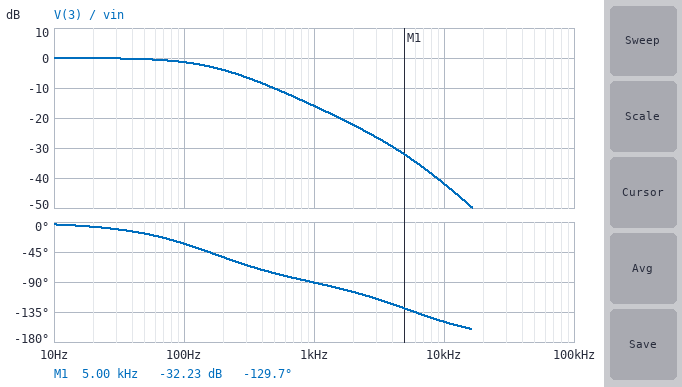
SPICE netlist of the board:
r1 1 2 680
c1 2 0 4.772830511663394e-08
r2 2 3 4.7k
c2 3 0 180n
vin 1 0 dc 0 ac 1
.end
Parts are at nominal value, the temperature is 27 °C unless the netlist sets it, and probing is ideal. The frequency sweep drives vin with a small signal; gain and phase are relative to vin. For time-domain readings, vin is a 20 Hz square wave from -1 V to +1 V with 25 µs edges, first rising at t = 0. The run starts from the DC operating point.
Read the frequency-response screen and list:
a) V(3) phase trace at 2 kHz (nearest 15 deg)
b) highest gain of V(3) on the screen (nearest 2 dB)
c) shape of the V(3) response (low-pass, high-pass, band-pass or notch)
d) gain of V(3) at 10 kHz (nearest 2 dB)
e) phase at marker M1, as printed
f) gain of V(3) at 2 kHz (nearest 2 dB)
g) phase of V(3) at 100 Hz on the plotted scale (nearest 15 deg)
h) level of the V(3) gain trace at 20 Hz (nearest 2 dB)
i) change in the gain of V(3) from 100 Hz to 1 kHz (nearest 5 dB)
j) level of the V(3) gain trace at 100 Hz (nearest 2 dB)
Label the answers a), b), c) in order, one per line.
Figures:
a) -105 deg
b) 0 dB
c) low-pass
d) -42 dB
e) -129.7 deg
f) -22 dB
g) -30 deg
h) 0 dB
i) -15 dB
j) -2 dB
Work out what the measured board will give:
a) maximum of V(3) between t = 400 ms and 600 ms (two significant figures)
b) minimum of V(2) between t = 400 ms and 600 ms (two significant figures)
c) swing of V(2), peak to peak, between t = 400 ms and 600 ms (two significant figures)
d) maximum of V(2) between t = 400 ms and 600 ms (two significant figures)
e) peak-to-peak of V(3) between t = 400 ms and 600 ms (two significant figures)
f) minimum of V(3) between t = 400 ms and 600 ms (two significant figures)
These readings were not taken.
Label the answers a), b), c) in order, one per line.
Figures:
a) 1.0 V
b) -1.0 V
c) 2.0 V
d) 1.0 V
e) 2.0 V
f) -1.0 V
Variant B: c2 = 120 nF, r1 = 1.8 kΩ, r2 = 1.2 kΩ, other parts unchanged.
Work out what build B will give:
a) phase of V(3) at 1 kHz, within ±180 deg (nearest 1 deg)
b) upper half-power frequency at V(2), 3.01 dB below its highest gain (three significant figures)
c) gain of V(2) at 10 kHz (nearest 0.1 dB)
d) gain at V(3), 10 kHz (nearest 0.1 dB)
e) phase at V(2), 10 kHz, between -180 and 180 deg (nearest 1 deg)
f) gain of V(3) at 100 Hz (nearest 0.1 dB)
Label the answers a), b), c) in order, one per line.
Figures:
a) -80 deg
b) 435 Hz
c) -15.7 dB
d) -34.9 dB
e) -66 deg
f) -0.3 dB
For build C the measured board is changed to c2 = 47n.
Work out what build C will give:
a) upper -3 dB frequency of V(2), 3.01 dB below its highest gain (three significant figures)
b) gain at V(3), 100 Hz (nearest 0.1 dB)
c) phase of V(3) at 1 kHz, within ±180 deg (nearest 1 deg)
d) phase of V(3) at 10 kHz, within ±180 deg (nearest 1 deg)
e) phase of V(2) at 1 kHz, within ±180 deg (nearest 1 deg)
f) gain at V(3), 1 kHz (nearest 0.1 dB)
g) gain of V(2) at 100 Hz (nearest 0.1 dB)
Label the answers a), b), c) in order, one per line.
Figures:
a) 3.98 kHz
b) -0.1 dB
c) -68 deg
d) -147 deg
e) -14 deg
f) -5.7 dB
g) 0 dB
